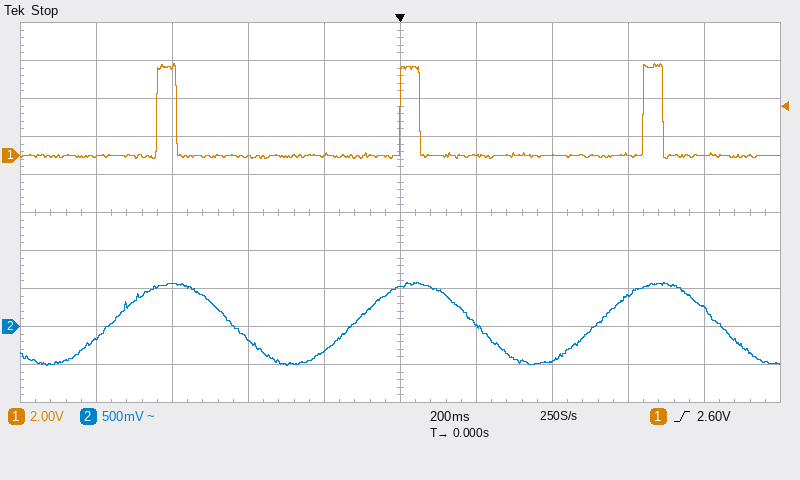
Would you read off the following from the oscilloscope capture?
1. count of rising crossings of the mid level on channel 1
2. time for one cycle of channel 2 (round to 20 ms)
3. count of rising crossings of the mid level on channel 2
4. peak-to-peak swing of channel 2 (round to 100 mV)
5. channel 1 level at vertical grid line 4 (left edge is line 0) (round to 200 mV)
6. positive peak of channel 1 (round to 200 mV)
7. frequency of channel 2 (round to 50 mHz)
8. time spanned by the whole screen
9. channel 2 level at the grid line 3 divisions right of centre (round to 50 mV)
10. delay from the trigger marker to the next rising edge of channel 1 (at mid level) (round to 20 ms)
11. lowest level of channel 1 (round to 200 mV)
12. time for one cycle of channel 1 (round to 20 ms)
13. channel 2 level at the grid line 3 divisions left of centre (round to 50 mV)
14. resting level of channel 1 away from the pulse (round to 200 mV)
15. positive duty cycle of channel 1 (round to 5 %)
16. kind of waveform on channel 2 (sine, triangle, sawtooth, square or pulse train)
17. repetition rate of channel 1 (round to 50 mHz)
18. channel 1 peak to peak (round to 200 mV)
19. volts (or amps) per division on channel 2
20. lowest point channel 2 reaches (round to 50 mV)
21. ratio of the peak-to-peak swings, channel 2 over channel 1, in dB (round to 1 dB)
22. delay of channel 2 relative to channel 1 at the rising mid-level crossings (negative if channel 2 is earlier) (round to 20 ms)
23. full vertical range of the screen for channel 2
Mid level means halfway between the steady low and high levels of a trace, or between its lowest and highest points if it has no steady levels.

3
640 ms
3
1.10 V
0.0 V
4.8 V
1.55 Hz
2 s
400 mV
640 ms
-200 mV
640 ms
550 mV
0.0 V
10 %
sine
1.55 Hz
5.0 V
500 mV
-500 mV
-13 dB
-120 ms
5 V
